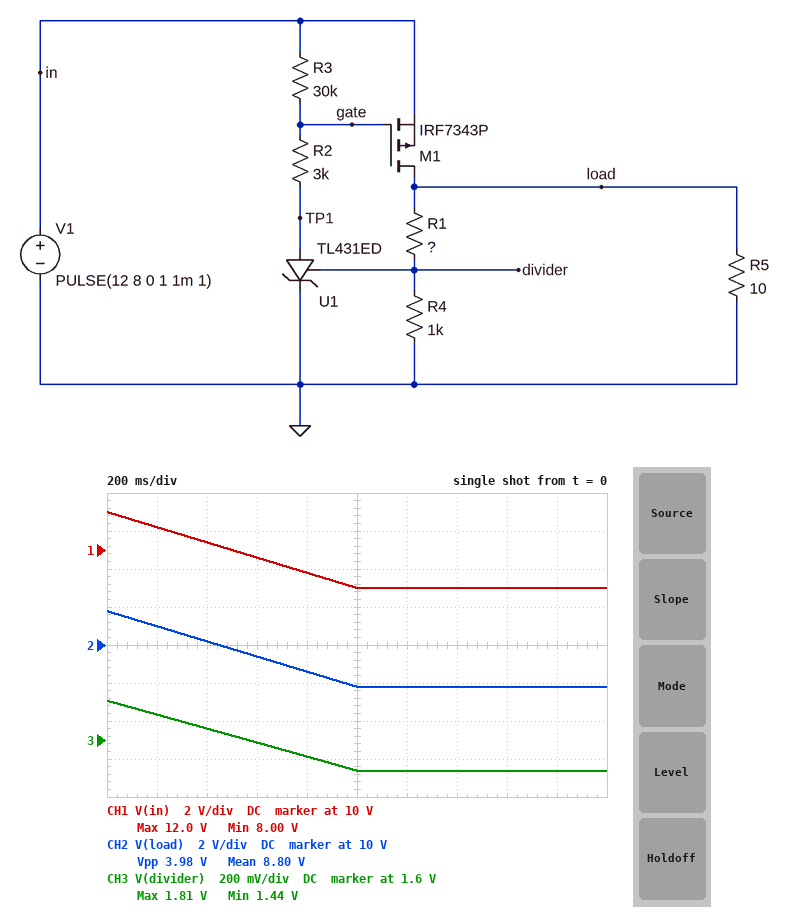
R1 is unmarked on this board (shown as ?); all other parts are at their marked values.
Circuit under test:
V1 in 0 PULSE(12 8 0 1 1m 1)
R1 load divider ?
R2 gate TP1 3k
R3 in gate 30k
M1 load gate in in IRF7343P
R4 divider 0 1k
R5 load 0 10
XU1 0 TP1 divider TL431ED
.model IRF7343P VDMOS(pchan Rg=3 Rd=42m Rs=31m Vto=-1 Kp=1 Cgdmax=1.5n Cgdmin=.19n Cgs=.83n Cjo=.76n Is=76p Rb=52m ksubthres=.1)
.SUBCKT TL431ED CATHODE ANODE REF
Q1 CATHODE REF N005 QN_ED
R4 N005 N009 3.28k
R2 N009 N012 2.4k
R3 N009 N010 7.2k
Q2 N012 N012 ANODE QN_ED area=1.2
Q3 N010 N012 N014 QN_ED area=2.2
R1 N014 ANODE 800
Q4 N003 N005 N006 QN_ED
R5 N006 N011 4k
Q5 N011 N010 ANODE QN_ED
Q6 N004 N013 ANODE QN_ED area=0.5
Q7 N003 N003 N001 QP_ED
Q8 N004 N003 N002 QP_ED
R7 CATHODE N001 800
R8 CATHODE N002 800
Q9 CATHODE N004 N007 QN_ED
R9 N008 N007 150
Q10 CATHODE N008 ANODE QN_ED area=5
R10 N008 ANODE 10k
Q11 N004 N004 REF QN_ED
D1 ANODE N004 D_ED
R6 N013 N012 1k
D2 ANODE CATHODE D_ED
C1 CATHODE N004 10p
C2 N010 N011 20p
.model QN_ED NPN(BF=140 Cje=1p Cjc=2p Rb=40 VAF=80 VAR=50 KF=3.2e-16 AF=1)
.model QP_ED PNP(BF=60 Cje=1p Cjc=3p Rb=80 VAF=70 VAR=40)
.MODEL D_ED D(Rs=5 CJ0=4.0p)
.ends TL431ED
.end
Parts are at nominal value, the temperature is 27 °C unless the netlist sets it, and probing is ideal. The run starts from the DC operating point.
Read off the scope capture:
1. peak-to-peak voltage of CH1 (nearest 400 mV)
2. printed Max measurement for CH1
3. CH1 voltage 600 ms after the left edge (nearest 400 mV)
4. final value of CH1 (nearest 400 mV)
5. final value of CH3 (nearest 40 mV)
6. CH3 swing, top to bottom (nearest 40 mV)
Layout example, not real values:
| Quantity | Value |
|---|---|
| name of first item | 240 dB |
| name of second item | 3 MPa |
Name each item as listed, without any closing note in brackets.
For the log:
| Quantity | Value |
|---|---|
| peak-to-peak voltage of CH1 | 4.0 V |
| printed Max measurement for CH1 | 12.0 V |
| CH1 voltage 600 ms after the left edge | 9.6 V |
| final value of CH1 | 8.0 V |
| final value of CH3 | 1.44 V |
| CH3 swing, top to bottom | 360 mV |
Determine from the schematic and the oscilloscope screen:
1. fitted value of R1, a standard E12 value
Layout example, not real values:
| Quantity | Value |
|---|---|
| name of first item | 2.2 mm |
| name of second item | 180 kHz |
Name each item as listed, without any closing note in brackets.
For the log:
| Quantity | Value |
|---|---|
| fitted value of R1, a standard E12 value | 390 Ω |
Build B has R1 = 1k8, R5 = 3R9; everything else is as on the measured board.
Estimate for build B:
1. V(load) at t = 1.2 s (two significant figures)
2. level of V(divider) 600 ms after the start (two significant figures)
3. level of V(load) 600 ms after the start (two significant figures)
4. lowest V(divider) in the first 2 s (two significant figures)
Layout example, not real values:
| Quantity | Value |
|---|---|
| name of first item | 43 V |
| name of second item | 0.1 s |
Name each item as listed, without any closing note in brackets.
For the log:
| Quantity | Value |
|---|---|
| V(load) at t = 1.2 s | 7.5 V |
| level of V(divider) 600 ms after the start | 950 mV |
| level of V(load) 600 ms after the start | 9.1 V |
| lowest V(divider) in the first 2 s | 910 mV |
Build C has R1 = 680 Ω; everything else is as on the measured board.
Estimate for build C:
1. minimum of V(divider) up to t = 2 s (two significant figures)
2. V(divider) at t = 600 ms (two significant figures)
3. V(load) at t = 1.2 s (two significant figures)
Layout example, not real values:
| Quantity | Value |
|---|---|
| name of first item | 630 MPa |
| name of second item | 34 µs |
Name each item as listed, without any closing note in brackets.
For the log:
| Quantity | Value |
|---|---|
| minimum of V(divider) up to t = 2 s | 1.2 V |
| V(divider) at t = 600 ms | 1.3 V |
| V(load) at t = 1.2 s | 7.8 V |
